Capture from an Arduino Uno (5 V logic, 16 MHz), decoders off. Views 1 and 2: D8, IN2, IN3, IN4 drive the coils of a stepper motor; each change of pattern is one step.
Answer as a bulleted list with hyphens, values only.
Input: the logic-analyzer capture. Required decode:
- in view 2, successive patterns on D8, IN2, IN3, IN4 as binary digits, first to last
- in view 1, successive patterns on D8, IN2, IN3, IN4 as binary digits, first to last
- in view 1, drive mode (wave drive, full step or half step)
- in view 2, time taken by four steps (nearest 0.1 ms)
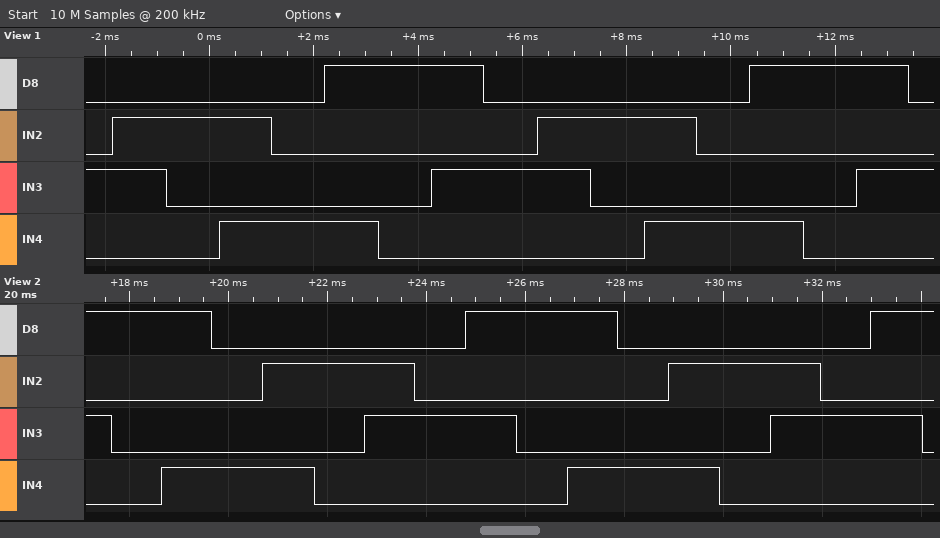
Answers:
- 1010 1000 1001 0001 0101 0100 0110 0010 1010 1000 1001 0001 0101 0100 0110 0010 1010 1000
- 0010 0110 0100 0101 0001 1001 1000 1010 0010 0110 0100 0101 0001 1001 1000 1010 0010
- half step
- 4.1 ms
